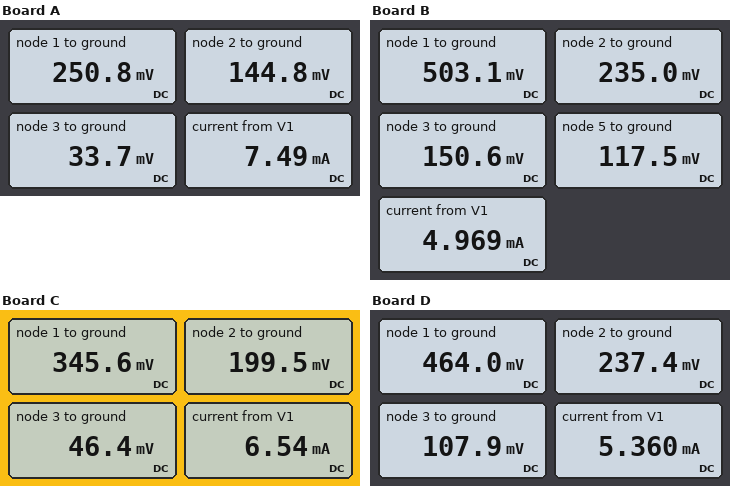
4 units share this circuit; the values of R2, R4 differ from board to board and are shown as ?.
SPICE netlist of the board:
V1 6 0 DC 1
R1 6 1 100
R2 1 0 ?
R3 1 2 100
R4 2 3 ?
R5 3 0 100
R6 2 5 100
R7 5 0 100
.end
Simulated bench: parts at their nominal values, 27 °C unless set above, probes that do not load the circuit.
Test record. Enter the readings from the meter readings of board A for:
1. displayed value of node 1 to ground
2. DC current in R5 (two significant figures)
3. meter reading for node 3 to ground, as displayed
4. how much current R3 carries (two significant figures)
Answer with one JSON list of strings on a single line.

["250.8 mV", "340 µA", "33.7 mV", "1.1 mA"]
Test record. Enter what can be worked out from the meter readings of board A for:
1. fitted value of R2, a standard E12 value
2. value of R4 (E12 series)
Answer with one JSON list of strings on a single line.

["39 Ω", "330 Ω"]
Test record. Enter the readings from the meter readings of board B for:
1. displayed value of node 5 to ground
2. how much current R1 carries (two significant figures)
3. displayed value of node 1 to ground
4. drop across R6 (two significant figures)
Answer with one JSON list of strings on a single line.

["117.5 mV", "5.0 mA", "503.1 mV", "120 mV"]
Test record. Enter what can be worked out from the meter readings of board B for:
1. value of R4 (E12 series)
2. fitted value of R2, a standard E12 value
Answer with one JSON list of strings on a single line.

["56 Ω", "220 Ω"]
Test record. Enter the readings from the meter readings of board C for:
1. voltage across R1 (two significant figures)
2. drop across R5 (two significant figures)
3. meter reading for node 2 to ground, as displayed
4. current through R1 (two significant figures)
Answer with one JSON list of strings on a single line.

["650 mV", "46 mV", "199.5 mV", "6.5 mA"]
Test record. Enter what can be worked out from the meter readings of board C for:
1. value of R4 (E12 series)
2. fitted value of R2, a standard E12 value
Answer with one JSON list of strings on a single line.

["330 Ω", "68 Ω"]
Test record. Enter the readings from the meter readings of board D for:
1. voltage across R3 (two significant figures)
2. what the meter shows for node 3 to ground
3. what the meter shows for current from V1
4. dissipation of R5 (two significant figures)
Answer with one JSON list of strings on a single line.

["230 mV", "107.9 mV", "5.360 mA", "120 µW"]
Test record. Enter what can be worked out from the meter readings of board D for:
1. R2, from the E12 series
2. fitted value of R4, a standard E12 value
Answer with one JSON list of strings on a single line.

["150 Ω", "120 Ω"]
